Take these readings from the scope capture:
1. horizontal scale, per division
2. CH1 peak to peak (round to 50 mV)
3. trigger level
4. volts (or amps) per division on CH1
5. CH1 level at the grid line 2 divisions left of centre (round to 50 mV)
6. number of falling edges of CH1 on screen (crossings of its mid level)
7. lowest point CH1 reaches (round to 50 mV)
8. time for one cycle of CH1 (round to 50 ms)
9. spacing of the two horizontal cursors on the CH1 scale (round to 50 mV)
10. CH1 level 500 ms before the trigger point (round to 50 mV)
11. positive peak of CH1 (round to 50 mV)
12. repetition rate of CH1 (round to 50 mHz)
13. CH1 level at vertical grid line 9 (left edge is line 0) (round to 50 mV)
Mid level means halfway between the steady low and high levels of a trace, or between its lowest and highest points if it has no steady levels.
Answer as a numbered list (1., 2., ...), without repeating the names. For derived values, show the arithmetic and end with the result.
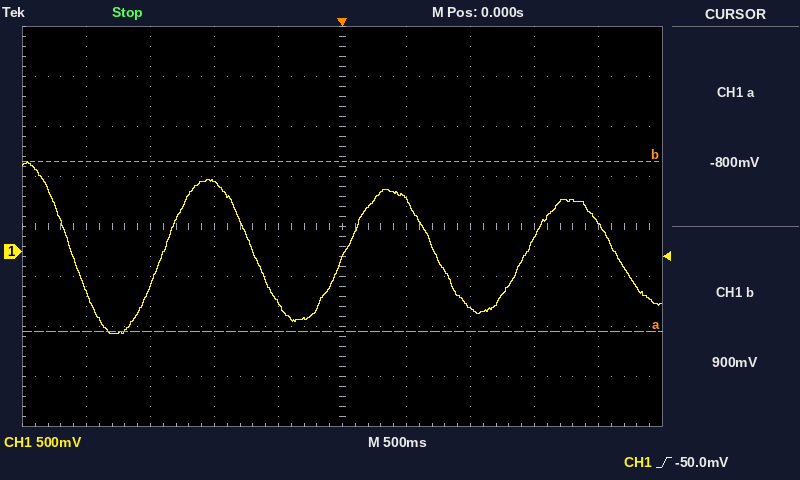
1. 500 ms
2. 900 mV − (-800 mV) = 1.70 V
3. -50.0 mV
4. 500 mV
5. 700 mV
6. 4
7. -800 mV
8. 1.40 s
9. 1.70 V
10. -500 mV
11. 900 mV
12. 1 / 1.40 s ≈ 714 mHz, so 700 mHz to the nearest 50 mHz
13. 300 mV
